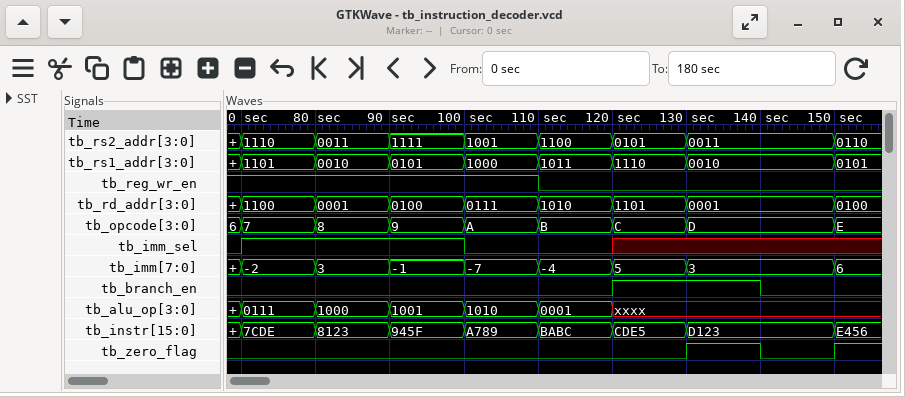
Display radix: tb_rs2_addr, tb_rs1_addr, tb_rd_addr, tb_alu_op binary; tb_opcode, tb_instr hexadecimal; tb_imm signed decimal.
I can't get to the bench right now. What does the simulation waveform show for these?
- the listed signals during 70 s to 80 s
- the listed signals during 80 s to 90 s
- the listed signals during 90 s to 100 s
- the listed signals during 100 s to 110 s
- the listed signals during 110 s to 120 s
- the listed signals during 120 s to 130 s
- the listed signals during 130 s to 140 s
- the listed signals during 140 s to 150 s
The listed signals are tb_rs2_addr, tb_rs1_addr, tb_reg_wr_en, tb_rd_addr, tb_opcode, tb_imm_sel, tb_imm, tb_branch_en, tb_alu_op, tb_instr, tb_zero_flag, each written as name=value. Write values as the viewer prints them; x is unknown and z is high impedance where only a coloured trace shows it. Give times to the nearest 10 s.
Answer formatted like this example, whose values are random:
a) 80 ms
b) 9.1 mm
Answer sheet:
a) tb_rs2_addr=1110, tb_rs1_addr=1101, tb_reg_wr_en=1, tb_rd_addr=1100, tb_opcode=7, tb_imm_sel=1, tb_imm=-2, tb_branch_en=0, tb_alu_op=0111, tb_instr=7CDE, tb_zero_flag=0
b) tb_rs2_addr=0011, tb_rs1_addr=0010, tb_reg_wr_en=1, tb_rd_addr=0001, tb_opcode=8, tb_imm_sel=1, tb_imm=3, tb_branch_en=0, tb_alu_op=1000, tb_instr=8123, tb_zero_flag=0
c) tb_rs2_addr=1111, tb_rs1_addr=0101, tb_reg_wr_en=1, tb_rd_addr=0100, tb_opcode=9, tb_imm_sel=1, tb_imm=-1, tb_branch_en=0, tb_alu_op=1001, tb_instr=945F, tb_zero_flag=0
d) tb_rs2_addr=1001, tb_rs1_addr=1000, tb_reg_wr_en=1, tb_rd_addr=0111, tb_opcode=A, tb_imm_sel=0, tb_imm=-7, tb_branch_en=0, tb_alu_op=1010, tb_instr=A789, tb_zero_flag=0
e) tb_rs2_addr=1100, tb_rs1_addr=1011, tb_reg_wr_en=0, tb_rd_addr=1010, tb_opcode=B, tb_imm_sel=0, tb_imm=-4, tb_branch_en=0, tb_alu_op=0001, tb_instr=BABC, tb_zero_flag=0
f) tb_rs2_addr=0101, tb_rs1_addr=1110, tb_reg_wr_en=0, tb_rd_addr=1101, tb_opcode=C, tb_imm_sel=x, tb_imm=5, tb_branch_en=1, tb_alu_op=xxxx, tb_instr=CDE5, tb_zero_flag=0
g) tb_rs2_addr=0011, tb_rs1_addr=0010, tb_reg_wr_en=0, tb_rd_addr=0001, tb_opcode=D, tb_imm_sel=x, tb_imm=3, tb_branch_en=1, tb_alu_op=xxxx, tb_instr=D123, tb_zero_flag=1
h) tb_rs2_addr=0011, tb_rs1_addr=0010, tb_reg_wr_en=0, tb_rd_addr=0001, tb_opcode=D, tb_imm_sel=x, tb_imm=3, tb_branch_en=0, tb_alu_op=xxxx, tb_instr=D123, tb_zero_flag=0
